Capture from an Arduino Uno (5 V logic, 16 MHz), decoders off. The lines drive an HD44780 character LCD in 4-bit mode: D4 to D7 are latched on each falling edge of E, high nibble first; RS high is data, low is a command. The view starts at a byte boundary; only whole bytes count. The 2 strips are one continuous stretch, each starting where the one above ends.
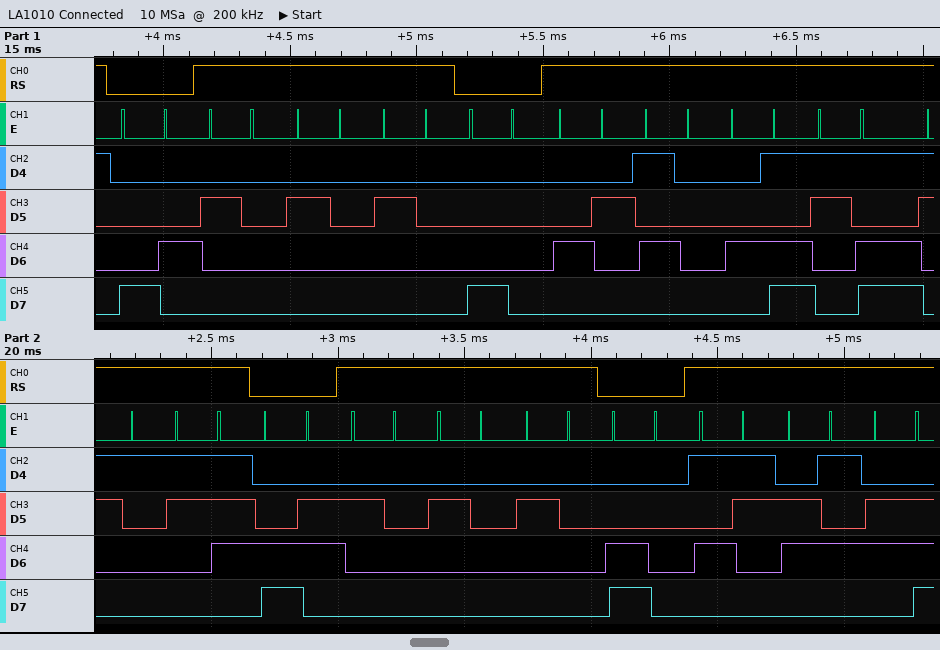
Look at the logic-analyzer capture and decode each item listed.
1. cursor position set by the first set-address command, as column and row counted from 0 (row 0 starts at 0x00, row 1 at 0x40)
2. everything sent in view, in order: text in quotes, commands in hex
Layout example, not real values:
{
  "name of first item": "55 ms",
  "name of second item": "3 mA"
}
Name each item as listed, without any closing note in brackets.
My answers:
{
  "cursor position set by the first set-address command, as column and row counted from 0": "column 4, row 0",
  "everything sent in view, in order: text in quotes, commands in hex": "0x84 \"   \" 0x80 \"BPM=17\" 0xC6 \"   \" 0xC0 \"Sen\""
}
